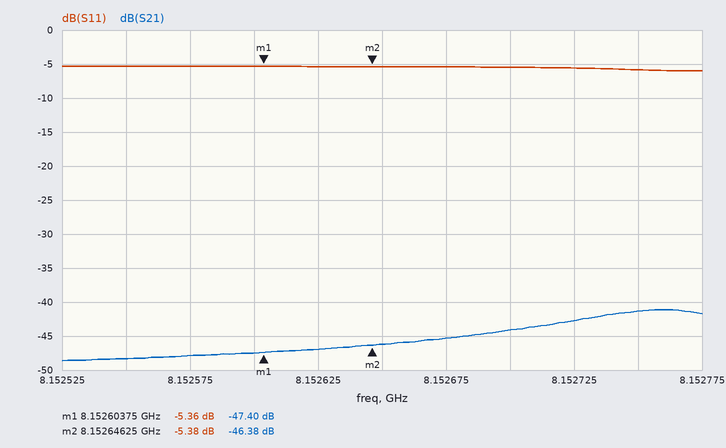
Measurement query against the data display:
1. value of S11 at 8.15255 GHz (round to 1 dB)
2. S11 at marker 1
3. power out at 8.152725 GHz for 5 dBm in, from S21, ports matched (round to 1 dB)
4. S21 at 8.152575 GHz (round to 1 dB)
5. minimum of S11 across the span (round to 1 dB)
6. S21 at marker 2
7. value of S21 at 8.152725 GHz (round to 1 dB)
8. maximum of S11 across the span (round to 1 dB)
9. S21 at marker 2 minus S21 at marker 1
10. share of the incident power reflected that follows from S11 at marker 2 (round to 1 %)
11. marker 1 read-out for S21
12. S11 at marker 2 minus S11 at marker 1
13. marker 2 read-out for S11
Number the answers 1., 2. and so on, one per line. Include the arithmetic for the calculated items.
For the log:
1. -5 dB
2. -5.36 dB
3. 5 dBm + (-43 dB) = -38 dBm
4. -48 dB
5. -6 dB
6. -46.38 dB
7. -43 dB
8. -5 dB
9. -46.38 − (-47.4) = 1.02 dB
10. 10^(-5.38/10) ≈ 29 %
11. -47.40 dB
12. -5.38 − (-5.36) = -0.02 dB
13. -5.38 dB
